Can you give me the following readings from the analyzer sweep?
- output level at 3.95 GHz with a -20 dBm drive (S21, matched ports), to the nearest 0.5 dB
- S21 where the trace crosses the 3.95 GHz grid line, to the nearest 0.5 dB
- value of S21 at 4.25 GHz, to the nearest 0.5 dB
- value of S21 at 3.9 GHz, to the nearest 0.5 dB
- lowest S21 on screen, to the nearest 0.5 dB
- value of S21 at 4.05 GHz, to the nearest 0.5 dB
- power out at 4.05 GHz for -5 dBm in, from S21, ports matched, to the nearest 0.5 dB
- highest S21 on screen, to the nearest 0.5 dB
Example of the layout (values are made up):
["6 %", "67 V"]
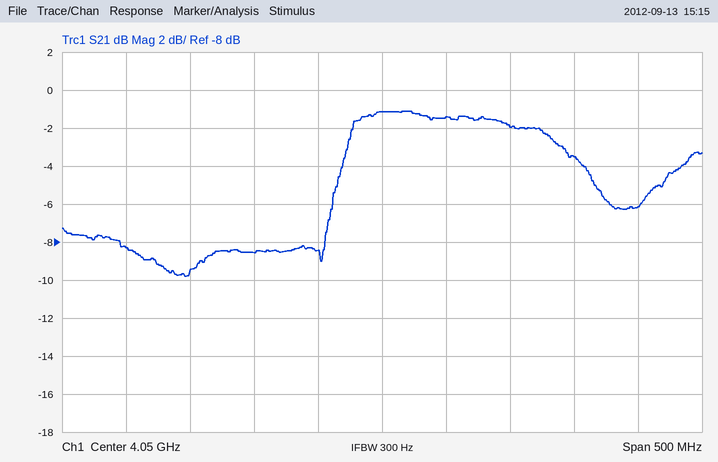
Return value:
["-28.5 dBm", "-8.5 dB", "-6.0 dB", "-9.5 dB", "-10.0 dB", "-1.0 dB", "-6.0 dBm", "-1.0 dB"]
